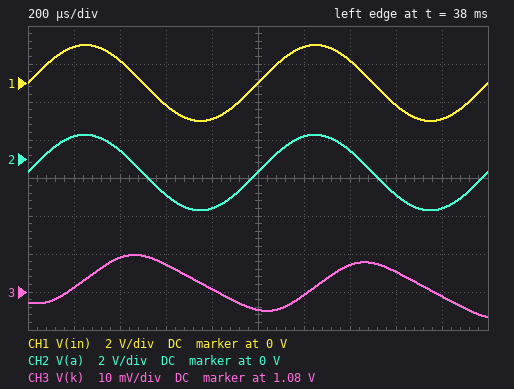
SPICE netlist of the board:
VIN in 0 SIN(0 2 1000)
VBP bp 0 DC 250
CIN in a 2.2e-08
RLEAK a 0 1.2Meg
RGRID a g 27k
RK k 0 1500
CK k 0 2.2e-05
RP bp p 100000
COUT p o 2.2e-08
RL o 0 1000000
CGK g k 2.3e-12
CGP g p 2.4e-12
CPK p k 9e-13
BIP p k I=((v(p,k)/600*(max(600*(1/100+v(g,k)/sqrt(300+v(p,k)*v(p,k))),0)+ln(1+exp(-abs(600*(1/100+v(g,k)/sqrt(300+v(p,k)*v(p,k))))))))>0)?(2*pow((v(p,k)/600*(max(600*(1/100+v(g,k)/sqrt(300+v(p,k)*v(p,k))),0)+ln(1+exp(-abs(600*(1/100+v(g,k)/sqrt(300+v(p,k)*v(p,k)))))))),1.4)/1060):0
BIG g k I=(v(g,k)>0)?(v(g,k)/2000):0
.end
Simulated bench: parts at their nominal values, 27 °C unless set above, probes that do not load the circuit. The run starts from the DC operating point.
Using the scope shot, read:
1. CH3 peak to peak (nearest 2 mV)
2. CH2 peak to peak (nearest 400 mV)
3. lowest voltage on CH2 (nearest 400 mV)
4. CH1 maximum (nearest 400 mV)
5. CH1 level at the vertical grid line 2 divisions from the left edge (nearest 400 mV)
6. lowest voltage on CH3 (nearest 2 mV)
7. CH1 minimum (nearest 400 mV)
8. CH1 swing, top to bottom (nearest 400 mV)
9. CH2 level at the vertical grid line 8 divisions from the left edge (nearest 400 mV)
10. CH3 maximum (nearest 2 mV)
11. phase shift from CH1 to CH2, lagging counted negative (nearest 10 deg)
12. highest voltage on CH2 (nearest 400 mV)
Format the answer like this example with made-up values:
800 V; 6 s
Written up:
16 mV; 4.0 V; -2.8 V; 2.0 V; 1.2 V; 1.074 V; -2.0 V; 4.0 V; -2.0 V; 1.090 V; 0 deg; 1.2 V
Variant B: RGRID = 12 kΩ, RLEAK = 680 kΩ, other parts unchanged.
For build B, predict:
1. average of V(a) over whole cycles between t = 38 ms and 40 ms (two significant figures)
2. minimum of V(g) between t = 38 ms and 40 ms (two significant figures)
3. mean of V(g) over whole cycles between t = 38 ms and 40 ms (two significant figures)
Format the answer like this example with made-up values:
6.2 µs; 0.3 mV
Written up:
-740 mV; -2.7 V; -750 mV
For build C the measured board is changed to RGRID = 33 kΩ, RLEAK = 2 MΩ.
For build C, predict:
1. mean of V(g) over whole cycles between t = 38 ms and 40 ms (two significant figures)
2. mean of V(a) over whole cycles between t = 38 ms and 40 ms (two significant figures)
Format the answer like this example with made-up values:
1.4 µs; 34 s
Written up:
-760 mV; -740 mV
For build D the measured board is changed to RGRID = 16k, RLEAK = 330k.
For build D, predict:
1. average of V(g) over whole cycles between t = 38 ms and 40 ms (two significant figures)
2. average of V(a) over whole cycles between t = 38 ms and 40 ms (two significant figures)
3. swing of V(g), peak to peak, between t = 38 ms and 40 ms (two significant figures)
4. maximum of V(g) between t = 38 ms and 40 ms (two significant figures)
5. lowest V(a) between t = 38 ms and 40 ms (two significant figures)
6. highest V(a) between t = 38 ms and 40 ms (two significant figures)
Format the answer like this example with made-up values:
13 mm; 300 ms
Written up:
-620 mV; -590 mV; 3.7 V; 1.1 V; -2.6 V; 1.4 V
